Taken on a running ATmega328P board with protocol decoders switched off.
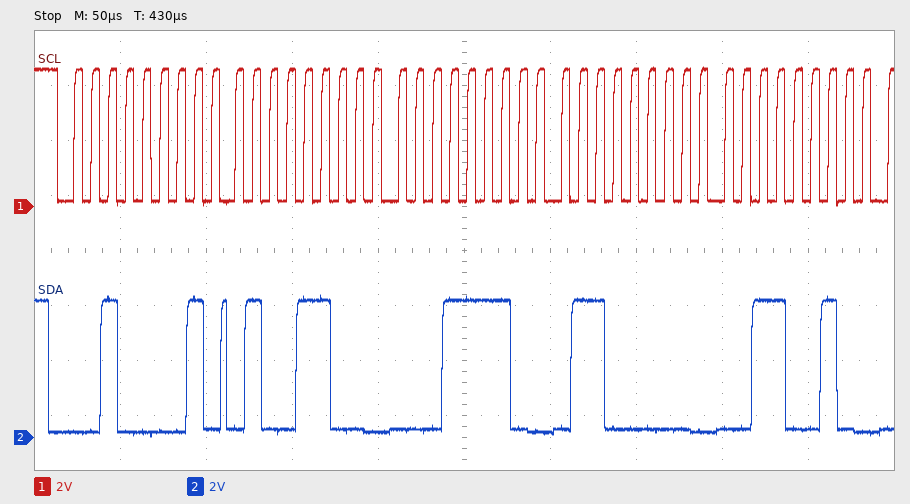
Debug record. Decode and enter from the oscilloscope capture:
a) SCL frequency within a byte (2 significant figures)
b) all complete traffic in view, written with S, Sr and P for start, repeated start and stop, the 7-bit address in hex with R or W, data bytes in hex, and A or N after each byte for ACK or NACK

100 kHz
S 10R A 4C A 1E A 60 A 32 A
